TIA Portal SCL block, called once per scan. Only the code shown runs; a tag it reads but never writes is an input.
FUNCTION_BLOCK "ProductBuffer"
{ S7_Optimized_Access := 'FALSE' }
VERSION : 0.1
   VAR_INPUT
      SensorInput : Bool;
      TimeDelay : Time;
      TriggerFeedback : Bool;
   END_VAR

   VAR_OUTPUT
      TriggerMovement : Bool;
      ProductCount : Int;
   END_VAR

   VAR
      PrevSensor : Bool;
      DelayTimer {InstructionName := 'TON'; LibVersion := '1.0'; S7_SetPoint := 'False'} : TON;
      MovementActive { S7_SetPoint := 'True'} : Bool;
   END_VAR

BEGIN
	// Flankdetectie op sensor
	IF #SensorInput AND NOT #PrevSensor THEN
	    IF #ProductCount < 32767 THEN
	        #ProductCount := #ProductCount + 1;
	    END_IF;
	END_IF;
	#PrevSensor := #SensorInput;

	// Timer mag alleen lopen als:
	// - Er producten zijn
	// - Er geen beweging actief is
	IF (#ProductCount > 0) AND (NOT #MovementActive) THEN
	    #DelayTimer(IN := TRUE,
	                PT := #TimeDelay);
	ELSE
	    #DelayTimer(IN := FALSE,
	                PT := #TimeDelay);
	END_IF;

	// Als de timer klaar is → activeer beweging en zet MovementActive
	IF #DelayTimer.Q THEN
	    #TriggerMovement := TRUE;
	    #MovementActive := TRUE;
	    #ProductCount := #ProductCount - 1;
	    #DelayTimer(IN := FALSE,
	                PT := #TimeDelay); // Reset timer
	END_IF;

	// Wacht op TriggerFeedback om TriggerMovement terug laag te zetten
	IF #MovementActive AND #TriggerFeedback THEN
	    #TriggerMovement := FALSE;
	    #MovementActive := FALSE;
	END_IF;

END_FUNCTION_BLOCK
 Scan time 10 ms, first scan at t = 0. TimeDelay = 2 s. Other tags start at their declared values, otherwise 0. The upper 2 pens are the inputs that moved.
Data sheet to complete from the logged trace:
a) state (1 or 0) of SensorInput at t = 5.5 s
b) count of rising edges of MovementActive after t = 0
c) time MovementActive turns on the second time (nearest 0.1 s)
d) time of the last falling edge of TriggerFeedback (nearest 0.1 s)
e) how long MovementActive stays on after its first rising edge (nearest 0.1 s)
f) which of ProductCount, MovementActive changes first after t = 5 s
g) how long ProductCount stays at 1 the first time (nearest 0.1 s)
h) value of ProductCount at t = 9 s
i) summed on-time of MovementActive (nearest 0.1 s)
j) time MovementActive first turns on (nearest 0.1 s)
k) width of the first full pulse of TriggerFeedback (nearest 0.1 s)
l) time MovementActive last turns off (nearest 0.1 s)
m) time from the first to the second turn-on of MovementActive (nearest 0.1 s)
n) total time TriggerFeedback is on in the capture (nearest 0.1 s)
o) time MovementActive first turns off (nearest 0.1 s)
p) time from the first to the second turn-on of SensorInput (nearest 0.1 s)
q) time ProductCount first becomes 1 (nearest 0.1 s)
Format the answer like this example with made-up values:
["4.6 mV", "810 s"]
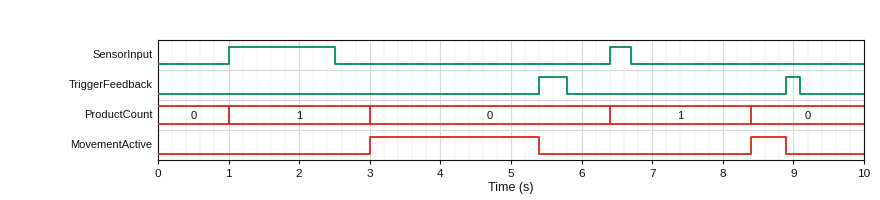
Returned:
["0", "2", "8.4 s", "9.1 s", "2.4 s", "MovementActive", "2.0 s", "0", "2.9 s", "3.0 s", "0.4 s", "8.9 s", "5.4 s", "0.6 s", "5.4 s", "5.4 s", "1.0 s"]
